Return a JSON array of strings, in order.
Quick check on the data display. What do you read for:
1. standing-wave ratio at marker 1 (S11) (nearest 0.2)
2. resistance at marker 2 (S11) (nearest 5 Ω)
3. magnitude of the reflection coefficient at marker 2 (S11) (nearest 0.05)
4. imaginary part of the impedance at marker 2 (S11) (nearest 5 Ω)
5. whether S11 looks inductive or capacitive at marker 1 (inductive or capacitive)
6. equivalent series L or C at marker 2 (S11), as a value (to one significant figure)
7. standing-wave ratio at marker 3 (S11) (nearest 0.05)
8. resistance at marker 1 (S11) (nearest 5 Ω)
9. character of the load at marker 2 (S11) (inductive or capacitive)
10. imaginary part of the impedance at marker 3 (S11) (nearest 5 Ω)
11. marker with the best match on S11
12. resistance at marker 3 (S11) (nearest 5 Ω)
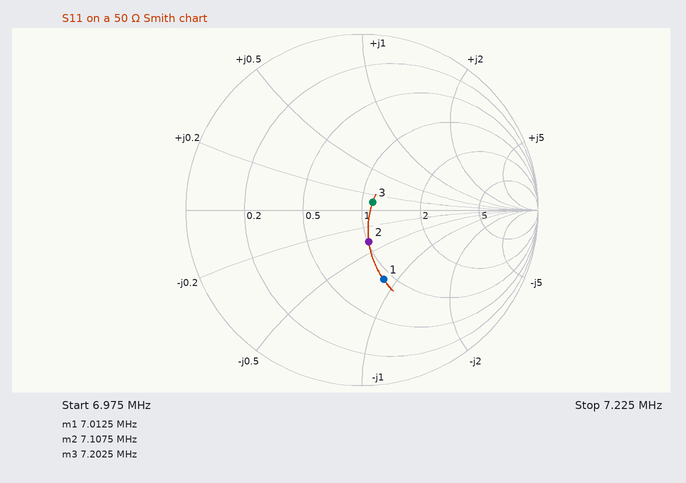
["2.4", "50 Ω", "0.20", "-20 Ω", "capacitive", "1 nF", "1.15", "45 Ω", "capacitive", "+5 Ω", "marker 3", "55 Ω"]
